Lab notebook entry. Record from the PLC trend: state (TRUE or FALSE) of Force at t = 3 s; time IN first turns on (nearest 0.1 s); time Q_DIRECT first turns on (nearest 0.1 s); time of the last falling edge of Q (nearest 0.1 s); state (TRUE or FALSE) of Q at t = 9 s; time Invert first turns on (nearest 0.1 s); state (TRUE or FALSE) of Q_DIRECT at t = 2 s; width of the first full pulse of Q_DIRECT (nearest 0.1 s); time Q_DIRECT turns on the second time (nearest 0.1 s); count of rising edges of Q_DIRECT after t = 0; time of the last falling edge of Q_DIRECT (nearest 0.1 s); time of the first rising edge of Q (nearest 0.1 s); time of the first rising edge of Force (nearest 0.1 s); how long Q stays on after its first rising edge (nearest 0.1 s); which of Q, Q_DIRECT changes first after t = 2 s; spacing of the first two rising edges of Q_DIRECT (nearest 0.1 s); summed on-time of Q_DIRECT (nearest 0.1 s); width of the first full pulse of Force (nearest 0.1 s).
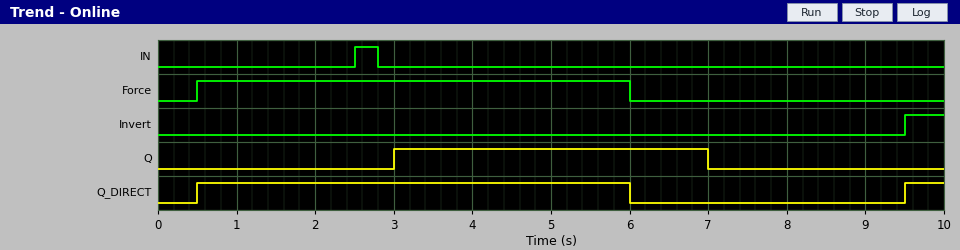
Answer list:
TRUE
2.5 s
0.5 s
7.0 s
FALSE
9.5 s
TRUE
5.5 s
9.5 s
2
6.0 s
3.0 s
0.5 s
4.0 s
Q
9.0 s
6.0 s
5.5 s
